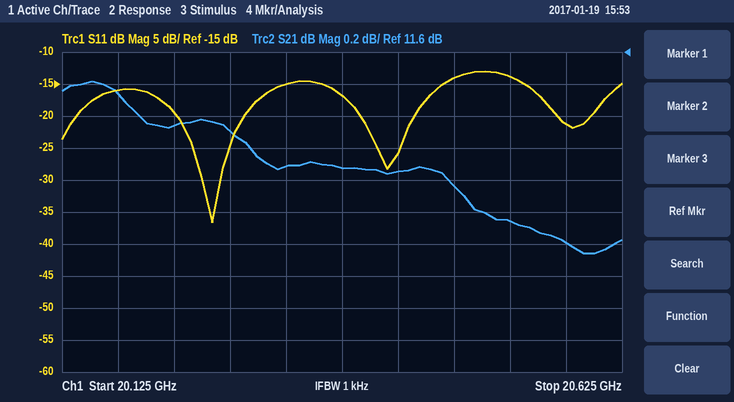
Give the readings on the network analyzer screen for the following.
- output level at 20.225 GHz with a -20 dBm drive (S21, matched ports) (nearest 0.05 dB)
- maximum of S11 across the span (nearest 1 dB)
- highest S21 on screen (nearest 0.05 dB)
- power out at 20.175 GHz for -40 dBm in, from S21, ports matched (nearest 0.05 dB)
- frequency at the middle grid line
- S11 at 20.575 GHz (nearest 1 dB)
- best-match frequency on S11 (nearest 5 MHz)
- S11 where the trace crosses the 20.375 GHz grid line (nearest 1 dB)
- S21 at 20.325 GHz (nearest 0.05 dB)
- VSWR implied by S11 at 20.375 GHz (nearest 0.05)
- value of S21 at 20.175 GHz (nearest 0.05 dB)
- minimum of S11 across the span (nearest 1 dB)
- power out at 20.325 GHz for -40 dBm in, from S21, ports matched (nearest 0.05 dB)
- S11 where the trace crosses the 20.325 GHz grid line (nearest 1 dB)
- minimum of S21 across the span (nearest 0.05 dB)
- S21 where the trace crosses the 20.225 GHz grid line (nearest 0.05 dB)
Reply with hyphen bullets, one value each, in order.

- -8.85 dBm
- -13 dB
- 11.40 dB
- -28.65 dBm
- 20.375 GHz
- -21 dB
- 20.260 GHz
- -17 dB
- 10.90 dB
- 1.35
- 11.35 dB
- -37 dB
- -29.10 dBm
- -15 dB
- 10.35 dB
- 11.15 dB
